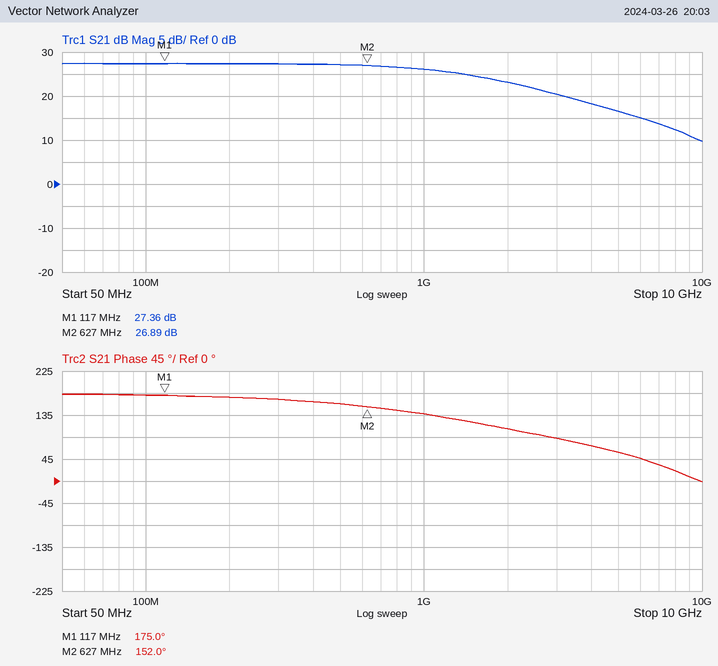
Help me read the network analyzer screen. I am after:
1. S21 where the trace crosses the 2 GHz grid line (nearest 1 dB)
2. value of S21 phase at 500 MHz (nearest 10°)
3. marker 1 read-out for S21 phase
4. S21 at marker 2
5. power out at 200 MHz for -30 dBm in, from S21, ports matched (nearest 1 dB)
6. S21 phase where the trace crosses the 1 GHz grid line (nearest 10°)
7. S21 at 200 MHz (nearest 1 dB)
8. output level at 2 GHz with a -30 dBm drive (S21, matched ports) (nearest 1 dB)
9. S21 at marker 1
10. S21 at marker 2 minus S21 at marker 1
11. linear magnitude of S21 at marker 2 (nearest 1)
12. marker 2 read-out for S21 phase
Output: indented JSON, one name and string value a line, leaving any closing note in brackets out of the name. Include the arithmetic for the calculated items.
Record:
{
  "S21 where the trace crosses the 2 GHz grid line": "23 dB",
  "value of S21 phase at 500 MHz": "160°",
  "marker 1 read-out for S21 phase": "175.0°",
  "S21 at marker 2": "26.89 dB",
  "power out at 200 MHz for -30 dBm in, from S21, ports matched": "-30 dBm + (27 dB) = -3 dBm",
  "S21 phase where the trace crosses the 1 GHz grid line": "140°",
  "S21 at 200 MHz": "27 dB",
  "output level at 2 GHz with a -30 dBm drive (S21, matched ports)": "-30 dBm + (23 dB) = -7 dBm",
  "S21 at marker 1": "27.36 dB",
  "S21 at marker 2 minus S21 at marker 1": "26.89 − (27.36) = -0.47 dB",
  "linear magnitude of S21 at marker 2": "10^(26.89/20) ≈ 22",
  "marker 2 read-out for S21 phase": "152.0°"
}
